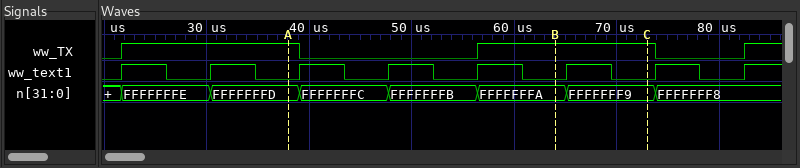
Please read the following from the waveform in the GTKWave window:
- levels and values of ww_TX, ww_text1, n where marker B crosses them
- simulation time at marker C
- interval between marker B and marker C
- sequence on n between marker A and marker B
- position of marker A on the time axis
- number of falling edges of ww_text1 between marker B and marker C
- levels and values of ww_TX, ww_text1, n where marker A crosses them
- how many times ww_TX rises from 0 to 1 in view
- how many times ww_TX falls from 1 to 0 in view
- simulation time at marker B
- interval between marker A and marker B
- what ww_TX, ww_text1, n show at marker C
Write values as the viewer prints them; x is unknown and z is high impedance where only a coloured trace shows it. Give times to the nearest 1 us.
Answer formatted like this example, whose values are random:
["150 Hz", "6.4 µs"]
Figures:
["ww_TX=1, ww_text1=0, n=FFFFFFFA", "73 us", "9 us", "FFFFFFFD, FFFFFFFC, FFFFFFFB, FFFFFFFA", "38 us", "1", "ww_TX=1, ww_text1=0, n=FFFFFFFD", "3", "2", "64 us", "26 us", "ww_TX=1, ww_text1=0, n=FFFFFFF9"]
